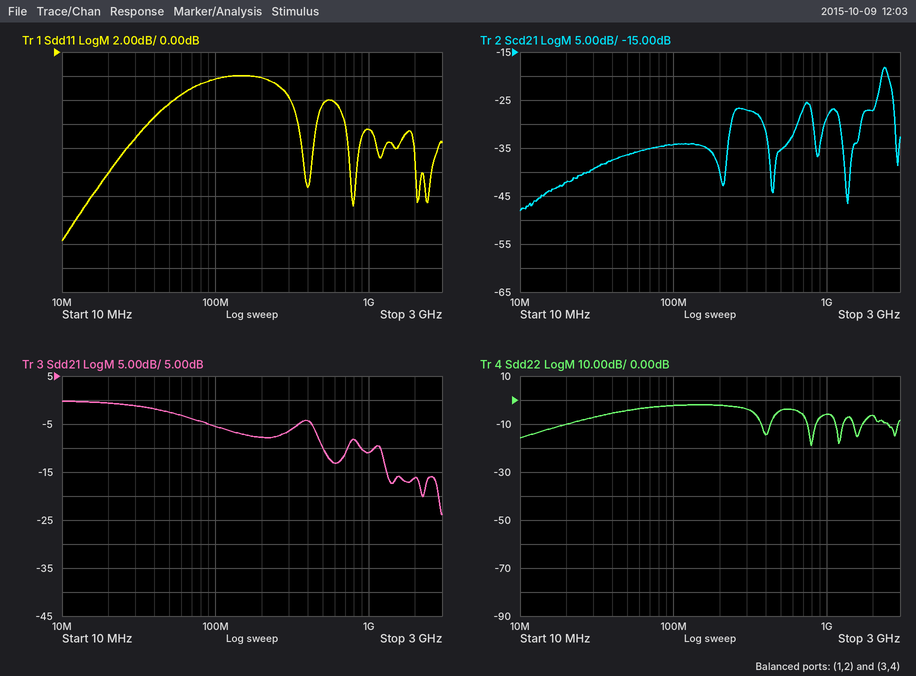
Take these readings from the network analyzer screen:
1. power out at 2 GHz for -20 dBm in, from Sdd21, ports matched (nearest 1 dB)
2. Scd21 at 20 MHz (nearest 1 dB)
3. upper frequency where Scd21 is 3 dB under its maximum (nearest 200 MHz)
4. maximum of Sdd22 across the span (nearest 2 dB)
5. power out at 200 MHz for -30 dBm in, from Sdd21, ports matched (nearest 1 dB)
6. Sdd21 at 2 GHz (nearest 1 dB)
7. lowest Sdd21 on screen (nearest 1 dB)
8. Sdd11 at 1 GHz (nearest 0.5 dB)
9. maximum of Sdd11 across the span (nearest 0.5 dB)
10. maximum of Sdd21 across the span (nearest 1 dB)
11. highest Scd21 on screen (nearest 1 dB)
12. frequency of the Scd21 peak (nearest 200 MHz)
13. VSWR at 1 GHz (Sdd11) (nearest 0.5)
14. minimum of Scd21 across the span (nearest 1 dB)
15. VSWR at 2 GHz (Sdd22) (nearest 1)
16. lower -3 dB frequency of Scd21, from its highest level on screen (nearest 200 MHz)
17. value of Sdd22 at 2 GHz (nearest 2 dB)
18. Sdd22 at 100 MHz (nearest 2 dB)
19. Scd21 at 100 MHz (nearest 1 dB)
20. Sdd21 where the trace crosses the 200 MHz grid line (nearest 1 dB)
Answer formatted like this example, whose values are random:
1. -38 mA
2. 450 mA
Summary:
1. -36 dBm
2. -42 dB
3. 2.6 GHz
4. -2 dB
5. -38 dBm
6. -16 dB
7. -24 dB
8. -6.5 dB
9. -2.0 dB
10. 0 dB
11. -18 dB
12. 2.4 GHz
13. 3.0
14. -48 dB
15. 3
16. 2.2 GHz
17. -6 dB
18. -2 dB
19. -34 dB
20. -8 dB
